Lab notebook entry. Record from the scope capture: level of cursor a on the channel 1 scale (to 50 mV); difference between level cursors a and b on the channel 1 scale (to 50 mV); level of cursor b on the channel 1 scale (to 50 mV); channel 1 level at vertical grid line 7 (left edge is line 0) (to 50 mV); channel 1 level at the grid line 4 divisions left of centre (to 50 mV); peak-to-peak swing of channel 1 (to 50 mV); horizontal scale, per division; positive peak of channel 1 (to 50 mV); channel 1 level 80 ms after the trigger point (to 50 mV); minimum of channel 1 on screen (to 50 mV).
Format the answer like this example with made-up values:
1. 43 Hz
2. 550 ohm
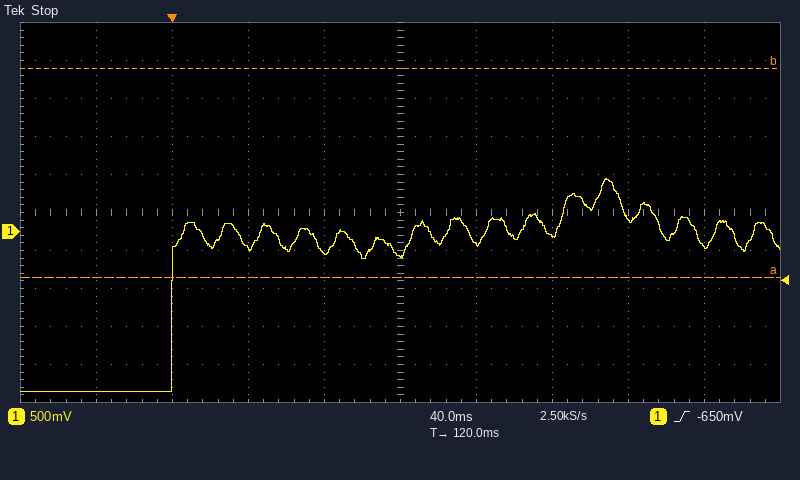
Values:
1. -600 mV
2. 2.75 V
3. 2.15 V
4. -50 mV
5. -2.10 V
6. 2.80 V
7. 40 ms
8. 700 mV
9. -250 mV
10. -2.10 V
